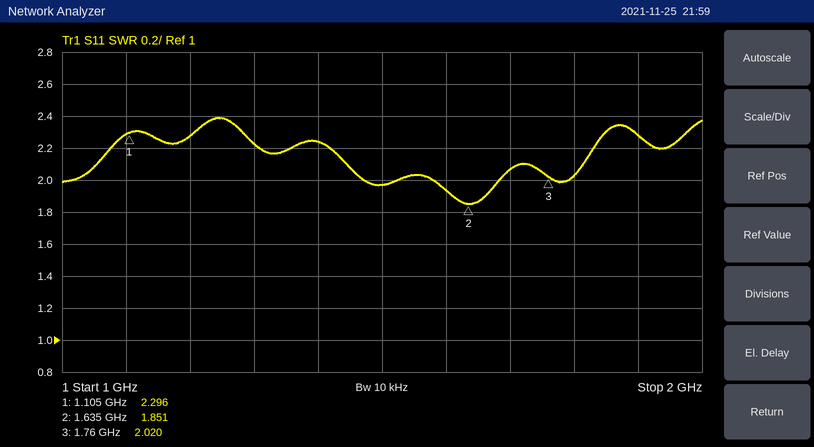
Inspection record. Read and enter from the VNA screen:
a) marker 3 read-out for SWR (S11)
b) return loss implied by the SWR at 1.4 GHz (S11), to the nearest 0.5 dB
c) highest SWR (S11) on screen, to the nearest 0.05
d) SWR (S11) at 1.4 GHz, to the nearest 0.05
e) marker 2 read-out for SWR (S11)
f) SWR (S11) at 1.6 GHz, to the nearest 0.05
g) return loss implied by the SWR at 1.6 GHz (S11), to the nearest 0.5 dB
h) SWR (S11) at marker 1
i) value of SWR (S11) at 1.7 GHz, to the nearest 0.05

2.020
8.5 dB
2.40
2.25
1.851
1.95
10.0 dB
2.296
2.05
